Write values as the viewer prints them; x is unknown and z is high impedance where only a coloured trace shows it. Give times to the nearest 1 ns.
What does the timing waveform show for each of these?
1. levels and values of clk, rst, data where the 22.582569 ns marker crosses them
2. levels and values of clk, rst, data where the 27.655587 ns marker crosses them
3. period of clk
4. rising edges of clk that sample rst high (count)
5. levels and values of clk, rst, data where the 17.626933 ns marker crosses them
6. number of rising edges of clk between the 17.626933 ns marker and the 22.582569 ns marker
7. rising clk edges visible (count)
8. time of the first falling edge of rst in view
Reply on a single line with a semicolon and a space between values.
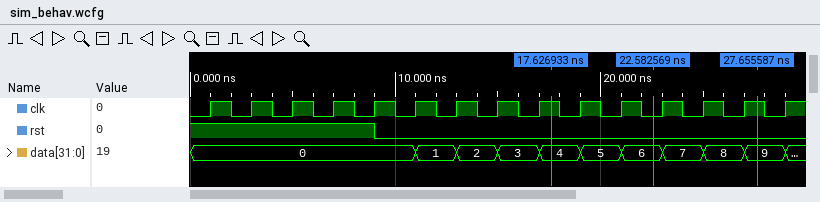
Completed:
clk=0, rst=0, data=6; clk=1, rst=0, data=9; 2 ns; 5; clk=1, rst=0, data=4; 2; 15; 9 ns
